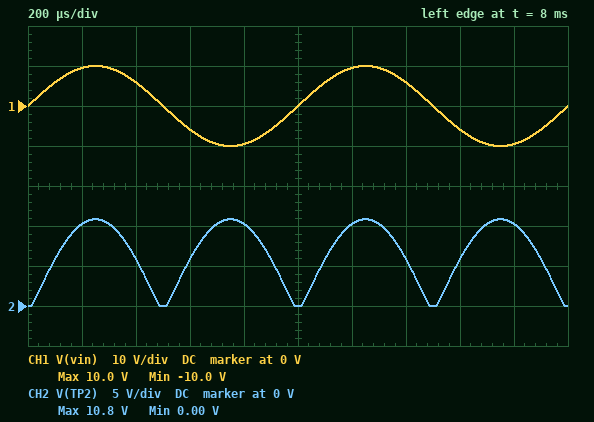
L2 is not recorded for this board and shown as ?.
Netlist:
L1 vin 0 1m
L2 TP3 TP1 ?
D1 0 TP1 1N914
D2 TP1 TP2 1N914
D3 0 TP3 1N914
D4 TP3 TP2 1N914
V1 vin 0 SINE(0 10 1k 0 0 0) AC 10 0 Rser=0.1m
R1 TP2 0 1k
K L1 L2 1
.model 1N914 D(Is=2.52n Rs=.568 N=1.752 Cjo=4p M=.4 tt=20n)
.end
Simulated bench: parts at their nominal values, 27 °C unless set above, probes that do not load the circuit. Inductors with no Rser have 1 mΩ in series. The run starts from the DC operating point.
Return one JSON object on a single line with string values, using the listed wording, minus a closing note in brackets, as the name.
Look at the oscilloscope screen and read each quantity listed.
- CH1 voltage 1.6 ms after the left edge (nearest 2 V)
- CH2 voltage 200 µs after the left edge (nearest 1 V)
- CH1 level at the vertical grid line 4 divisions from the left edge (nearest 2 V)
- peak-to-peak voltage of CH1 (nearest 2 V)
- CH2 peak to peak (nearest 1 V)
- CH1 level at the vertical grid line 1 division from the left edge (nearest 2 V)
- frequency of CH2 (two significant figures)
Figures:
{"CH1 voltage 1.6 ms after the left edge": "-6 V", "CH2 voltage 200 µs after the left edge": "10 V", "CH1 level at the vertical grid line 4 divisions from the left edge": "-10 V", "peak-to-peak voltage of CH1": "20 V", "CH2 peak to peak": "11 V", "CH1 level at the vertical grid line 1 division from the left edge": "10 V", "frequency of CH2": "2.0 kHz"}
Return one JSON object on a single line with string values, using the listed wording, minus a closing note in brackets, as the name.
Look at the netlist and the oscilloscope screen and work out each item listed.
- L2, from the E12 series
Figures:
{"L2, from the E12 series": "1.5 mH"}
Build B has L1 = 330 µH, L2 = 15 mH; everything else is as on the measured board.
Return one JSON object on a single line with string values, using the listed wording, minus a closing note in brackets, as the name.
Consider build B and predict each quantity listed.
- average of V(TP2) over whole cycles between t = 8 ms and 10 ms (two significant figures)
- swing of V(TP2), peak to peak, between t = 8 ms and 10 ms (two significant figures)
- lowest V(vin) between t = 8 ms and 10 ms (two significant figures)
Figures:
{"average of V(TP2) over whole cycles between t = 8 ms and 10 ms": "41 V", "swing of V(TP2), peak to peak, between t = 8 ms and 10 ms": "66 V", "lowest V(vin) between t = 8 ms and 10 ms": "-10 V"}
